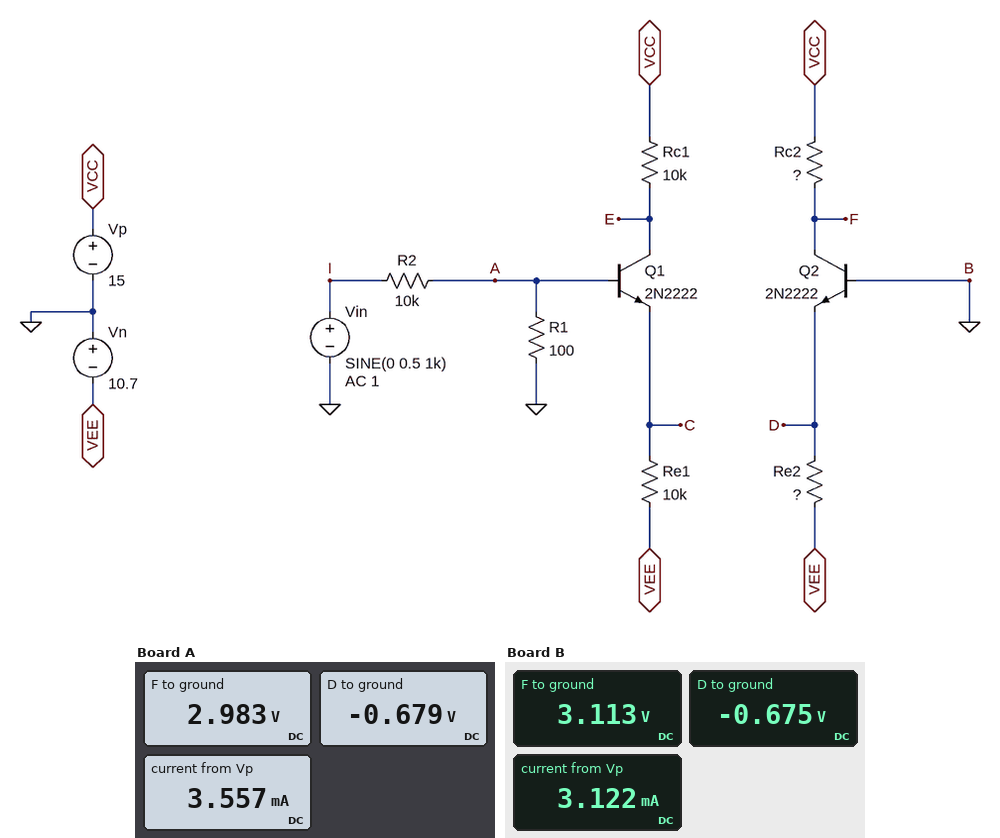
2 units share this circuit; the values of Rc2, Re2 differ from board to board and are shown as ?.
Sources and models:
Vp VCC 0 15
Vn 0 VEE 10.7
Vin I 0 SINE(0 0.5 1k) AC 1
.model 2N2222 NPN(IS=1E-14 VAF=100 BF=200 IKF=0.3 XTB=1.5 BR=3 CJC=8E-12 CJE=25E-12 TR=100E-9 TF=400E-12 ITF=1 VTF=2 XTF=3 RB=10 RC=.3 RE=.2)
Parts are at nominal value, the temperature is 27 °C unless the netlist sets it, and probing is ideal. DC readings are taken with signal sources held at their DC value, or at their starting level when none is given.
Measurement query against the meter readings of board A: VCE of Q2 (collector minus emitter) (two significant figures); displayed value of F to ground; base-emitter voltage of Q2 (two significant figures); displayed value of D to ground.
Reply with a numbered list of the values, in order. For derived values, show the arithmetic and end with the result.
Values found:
1. 2.983 V - (-679 mV) = 3.7 V
2. 2.983 V
3. 0 V - (-679 mV) = 680 mV
4. -0.679 V
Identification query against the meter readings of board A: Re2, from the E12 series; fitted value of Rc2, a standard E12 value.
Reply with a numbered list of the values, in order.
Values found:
1. 3.9 kΩ
2. 4.7 kΩ
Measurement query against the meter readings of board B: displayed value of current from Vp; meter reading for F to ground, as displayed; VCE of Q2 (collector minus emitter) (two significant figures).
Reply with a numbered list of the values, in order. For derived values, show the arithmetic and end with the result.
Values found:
1. 3.122 mA
2. 3.113 V
3. 3.113 V - (-675 mV) = 3.8 V
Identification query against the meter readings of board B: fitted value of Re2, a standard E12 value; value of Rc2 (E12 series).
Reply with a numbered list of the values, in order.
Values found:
1. 4.7 kΩ
2. 5.6 kΩ
